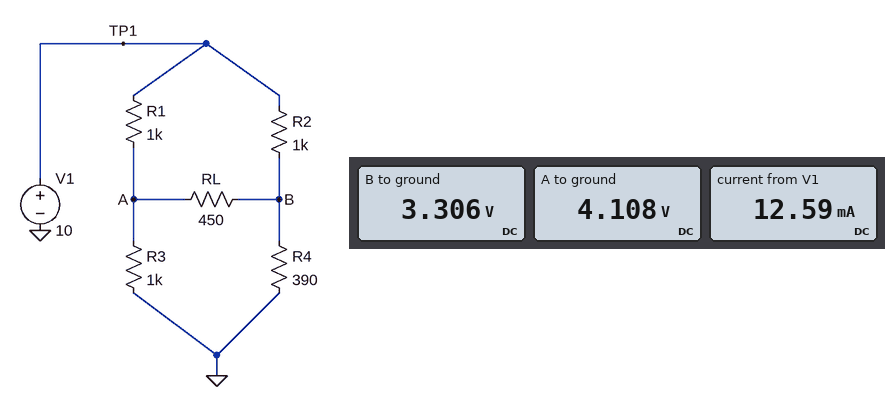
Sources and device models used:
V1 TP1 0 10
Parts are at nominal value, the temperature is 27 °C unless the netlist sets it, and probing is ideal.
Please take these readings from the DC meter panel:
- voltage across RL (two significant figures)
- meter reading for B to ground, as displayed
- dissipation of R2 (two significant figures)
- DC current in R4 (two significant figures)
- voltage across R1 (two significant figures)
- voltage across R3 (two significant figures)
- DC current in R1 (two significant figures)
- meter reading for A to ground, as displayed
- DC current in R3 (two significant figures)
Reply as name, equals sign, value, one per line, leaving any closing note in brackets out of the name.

voltage across RL = 800 mV
meter reading for B to ground, as displayed = 3.306 V
dissipation of R2 = 45 mW
DC current in R4 = 8.5 mA
voltage across R1 = 5.9 V
voltage across R3 = 4.1 V
DC current in R1 = 5.9 mA
meter reading for A to ground, as displayed = 4.108 V
DC current in R3 = 4.1 mA
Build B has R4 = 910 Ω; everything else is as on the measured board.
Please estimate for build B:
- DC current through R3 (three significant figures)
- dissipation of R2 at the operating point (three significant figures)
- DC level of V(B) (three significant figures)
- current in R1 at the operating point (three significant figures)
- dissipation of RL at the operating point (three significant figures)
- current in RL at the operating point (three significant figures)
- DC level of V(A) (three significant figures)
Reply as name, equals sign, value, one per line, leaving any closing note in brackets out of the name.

DC current through R3 = 4.92 mA
dissipation of R2 at the operating point = 26.6 mW
DC level of V(B) = 4.84 V
current in R1 at the operating point = 5.08 mA
dissipation of RL at the operating point = 12.3 µW
current in RL at the operating point = 165 µA
DC level of V(A) = 4.92 V
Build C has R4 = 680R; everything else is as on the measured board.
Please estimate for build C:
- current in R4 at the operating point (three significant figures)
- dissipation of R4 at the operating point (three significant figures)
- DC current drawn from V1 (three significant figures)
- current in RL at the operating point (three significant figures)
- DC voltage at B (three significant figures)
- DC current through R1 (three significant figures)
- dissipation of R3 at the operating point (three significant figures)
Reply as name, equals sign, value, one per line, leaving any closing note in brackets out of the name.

current in R4 at the operating point = 6.37 mA
dissipation of R4 at the operating point = 27.6 mW
DC current drawn from V1 = 11.0 mA
current in RL at the operating point = 703 µA
DC voltage at B = 4.33 V
DC current through R1 = 5.35 mA
dissipation of R3 at the operating point = 21.6 mW
